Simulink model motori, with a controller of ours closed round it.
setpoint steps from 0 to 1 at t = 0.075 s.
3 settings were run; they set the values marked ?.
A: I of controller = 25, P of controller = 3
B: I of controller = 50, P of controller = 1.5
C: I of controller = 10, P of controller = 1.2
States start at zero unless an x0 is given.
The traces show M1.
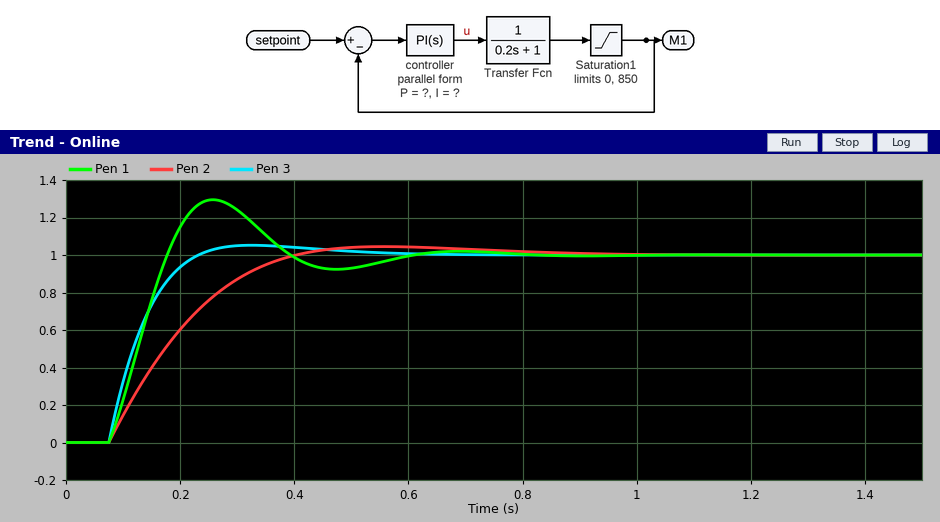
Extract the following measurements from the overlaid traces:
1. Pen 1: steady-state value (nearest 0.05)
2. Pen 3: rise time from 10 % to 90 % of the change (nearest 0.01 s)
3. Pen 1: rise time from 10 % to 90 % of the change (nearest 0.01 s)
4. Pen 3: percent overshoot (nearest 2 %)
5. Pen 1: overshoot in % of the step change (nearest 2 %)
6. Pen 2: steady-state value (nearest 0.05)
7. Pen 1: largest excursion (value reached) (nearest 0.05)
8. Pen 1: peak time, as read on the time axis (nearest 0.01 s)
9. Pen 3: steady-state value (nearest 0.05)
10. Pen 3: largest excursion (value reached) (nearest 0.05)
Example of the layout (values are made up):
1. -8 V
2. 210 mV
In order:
1. 1.00
2. 0.11 s
3. 0.08 s
4. 6 %
5. 30 %
6. 1.00
7. 1.30
8. 0.26 s
9. 1.00
10. 1.05
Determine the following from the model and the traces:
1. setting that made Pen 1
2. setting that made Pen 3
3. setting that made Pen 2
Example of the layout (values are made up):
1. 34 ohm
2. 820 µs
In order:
1. B
2. A
3. C
